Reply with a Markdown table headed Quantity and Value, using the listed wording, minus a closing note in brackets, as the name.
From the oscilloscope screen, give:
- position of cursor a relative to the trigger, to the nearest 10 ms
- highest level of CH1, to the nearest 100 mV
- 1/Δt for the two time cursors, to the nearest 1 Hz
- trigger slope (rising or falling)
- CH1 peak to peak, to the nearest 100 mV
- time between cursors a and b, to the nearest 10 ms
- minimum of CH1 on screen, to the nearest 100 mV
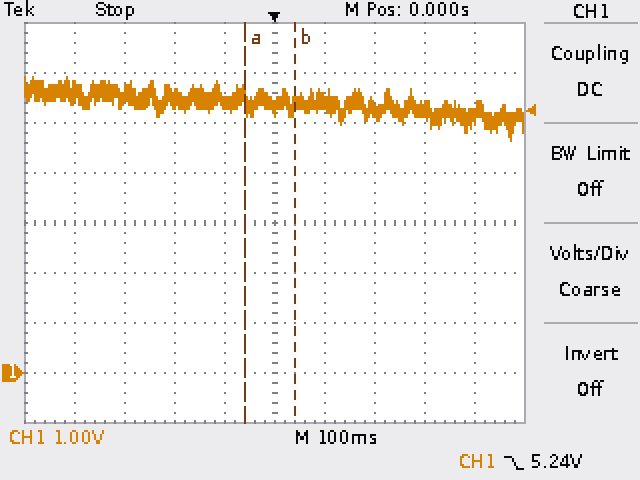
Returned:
| Quantity | Value |
|---|---|
| position of cursor a relative to the trigger, to the nearest 10 ms | -60 ms |
| highest level of CH1, to the nearest 100 mV | 5.9 V |
| 1/Δt for the two time cursors, to the nearest 1 Hz | 10 Hz |
| trigger slope | falling |
| CH1 peak to peak, to the nearest 100 mV | 1.3 V |
| time between cursors a and b, to the nearest 10 ms | 100 ms |
| minimum of CH1 on screen, to the nearest 100 mV | 4.6 V |
